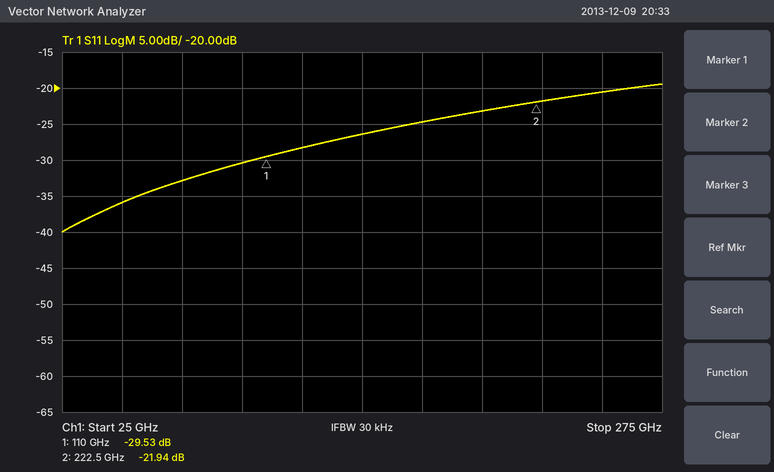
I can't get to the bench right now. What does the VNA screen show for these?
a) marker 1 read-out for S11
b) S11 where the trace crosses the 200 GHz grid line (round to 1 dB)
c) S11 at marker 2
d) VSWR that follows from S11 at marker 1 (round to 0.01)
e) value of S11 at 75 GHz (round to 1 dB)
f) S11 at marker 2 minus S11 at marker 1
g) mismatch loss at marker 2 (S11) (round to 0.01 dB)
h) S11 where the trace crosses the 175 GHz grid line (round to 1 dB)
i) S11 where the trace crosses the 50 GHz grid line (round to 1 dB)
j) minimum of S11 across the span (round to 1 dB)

-29.53 dB
-23 dB
-21.94 dB
1.07
-33 dB
7.59 dB
0.03 dB
-25 dB
-36 dB
-40 dB
